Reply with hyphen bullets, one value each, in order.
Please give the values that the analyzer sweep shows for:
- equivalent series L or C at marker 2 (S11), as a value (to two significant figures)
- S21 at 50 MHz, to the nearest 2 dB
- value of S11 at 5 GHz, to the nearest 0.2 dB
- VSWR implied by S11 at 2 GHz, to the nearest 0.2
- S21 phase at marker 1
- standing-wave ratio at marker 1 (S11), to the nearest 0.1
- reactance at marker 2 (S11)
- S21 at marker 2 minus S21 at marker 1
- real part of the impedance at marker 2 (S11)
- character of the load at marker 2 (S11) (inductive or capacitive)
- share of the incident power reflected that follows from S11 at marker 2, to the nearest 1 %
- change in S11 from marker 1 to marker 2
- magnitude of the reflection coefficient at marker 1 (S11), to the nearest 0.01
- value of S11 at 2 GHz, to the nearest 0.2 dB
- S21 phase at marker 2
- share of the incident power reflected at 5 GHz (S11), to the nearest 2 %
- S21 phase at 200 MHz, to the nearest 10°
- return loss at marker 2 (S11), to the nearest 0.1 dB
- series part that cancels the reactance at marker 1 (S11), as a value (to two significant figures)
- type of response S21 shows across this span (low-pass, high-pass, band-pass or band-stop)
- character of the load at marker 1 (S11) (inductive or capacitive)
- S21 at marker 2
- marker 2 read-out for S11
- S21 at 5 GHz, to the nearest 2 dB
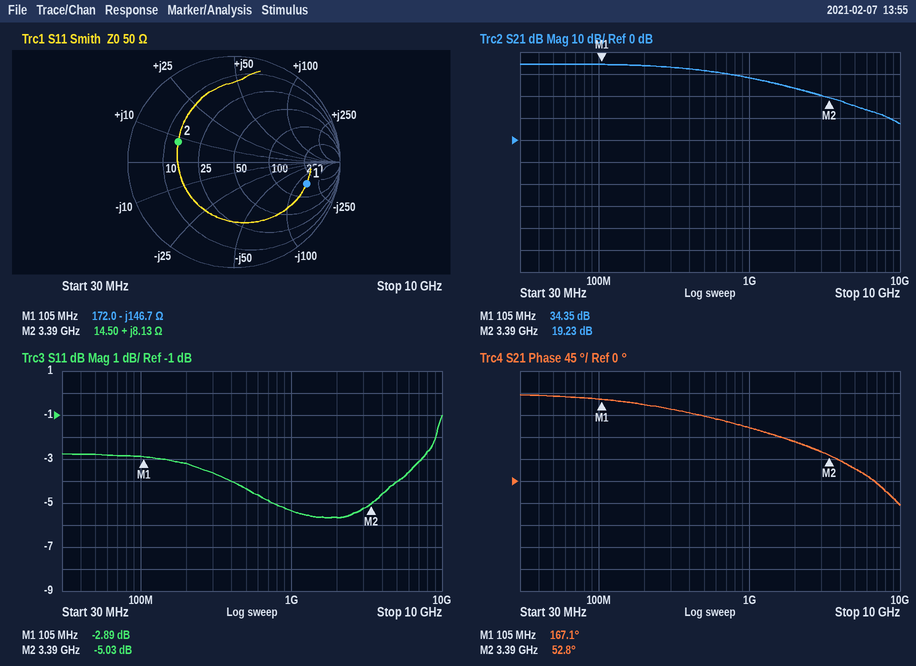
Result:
- 380 pH
- 34 dB
- -4.0 dB
- 3.2
- 167.1°
- 6.1
- +8.13 Ω
- -15.12 dB
- 14.50 Ω
- inductive
- 31 %
- -2.14 dB
- 0.72
- -5.6 dB
- 52.8°
- 40 %
- 160°
- 5.0 dB
- 220 nH
- low-pass
- capacitive
- 19.23 dB
- -5.03 dB
- 16 dB
